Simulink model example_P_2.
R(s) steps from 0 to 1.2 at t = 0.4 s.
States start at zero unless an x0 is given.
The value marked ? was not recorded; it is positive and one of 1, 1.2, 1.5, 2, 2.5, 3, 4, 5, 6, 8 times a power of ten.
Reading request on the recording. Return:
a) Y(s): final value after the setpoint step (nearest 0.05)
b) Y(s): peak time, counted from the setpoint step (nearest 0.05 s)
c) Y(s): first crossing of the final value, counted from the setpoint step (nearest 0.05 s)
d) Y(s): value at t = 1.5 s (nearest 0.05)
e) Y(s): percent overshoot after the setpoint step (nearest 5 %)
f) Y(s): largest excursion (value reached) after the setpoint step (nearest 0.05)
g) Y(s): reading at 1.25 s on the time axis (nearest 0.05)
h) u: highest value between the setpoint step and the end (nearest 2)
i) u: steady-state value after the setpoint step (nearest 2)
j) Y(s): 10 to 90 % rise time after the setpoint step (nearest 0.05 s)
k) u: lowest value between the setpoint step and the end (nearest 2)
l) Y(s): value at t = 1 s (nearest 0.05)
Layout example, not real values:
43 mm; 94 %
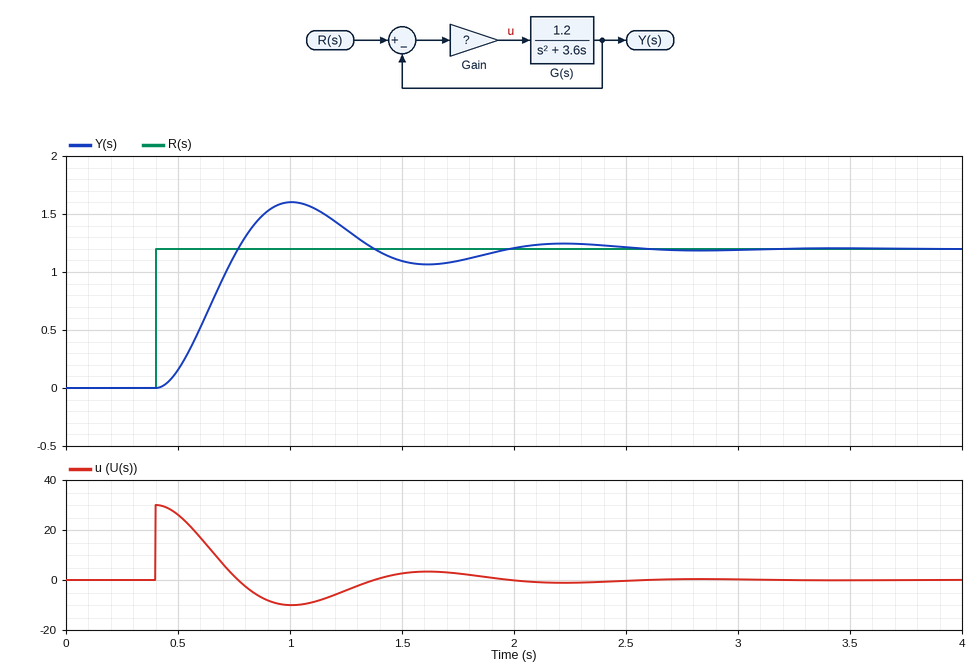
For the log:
1.20; 0.60 s; 0.35 s; 1.10; 35 %; 1.60; 1.35; 30; 0; 0.25 s; -10; 1.60
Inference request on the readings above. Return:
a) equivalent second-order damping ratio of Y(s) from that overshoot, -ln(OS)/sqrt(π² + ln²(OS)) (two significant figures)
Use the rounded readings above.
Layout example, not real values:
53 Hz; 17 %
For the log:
0.32
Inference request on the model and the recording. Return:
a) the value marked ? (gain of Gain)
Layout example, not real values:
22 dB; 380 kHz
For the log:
25
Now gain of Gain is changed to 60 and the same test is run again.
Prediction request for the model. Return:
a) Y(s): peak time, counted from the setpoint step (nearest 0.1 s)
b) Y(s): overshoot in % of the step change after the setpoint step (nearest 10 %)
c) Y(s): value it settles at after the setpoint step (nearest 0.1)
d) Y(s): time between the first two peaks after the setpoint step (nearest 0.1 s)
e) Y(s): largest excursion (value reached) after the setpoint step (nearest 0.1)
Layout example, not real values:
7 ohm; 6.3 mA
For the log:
0.4 s; 50 %; 1.2; 0.8 s; 1.8
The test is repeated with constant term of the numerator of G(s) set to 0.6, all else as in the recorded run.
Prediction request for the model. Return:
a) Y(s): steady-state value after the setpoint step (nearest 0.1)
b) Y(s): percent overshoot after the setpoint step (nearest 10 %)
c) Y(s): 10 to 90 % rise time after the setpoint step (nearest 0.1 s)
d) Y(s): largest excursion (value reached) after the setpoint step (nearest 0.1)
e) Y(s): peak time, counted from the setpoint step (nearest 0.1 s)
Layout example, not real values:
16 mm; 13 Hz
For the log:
1.2; 20 %; 0.4 s; 1.4; 0.9 s
